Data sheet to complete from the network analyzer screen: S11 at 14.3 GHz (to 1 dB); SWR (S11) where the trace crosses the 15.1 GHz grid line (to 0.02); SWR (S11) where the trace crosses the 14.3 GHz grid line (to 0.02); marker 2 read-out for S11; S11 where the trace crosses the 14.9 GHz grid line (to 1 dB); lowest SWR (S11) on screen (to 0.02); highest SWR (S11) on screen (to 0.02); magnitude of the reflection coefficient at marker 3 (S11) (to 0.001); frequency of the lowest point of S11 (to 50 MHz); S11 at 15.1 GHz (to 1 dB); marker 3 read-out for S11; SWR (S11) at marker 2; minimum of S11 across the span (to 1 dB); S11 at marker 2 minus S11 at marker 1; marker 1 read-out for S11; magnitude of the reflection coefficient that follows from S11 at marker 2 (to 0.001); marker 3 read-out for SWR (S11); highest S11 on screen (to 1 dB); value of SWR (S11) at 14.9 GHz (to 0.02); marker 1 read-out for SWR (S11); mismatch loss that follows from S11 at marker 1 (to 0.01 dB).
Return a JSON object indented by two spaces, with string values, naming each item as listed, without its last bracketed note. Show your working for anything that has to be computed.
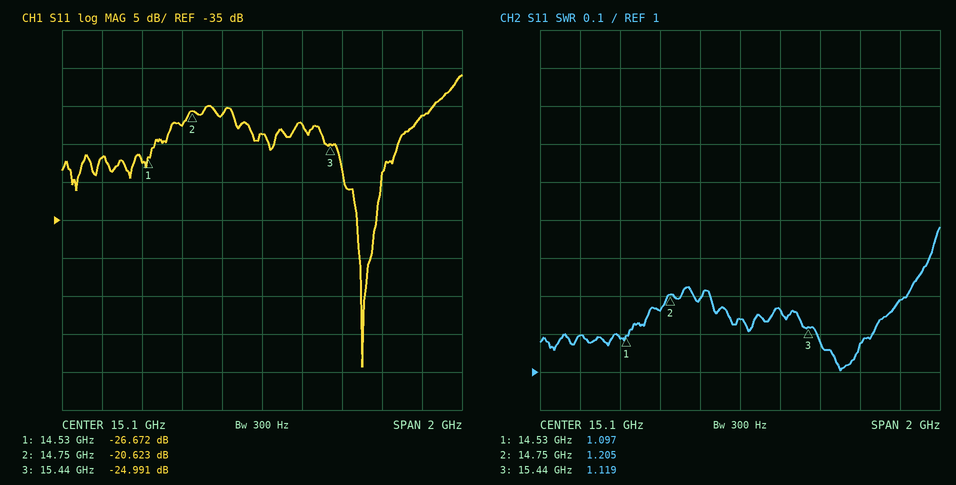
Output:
{
  "S11 at 14.3 GHz": "-27 dB",
  "SWR (S11) where the trace crosses the 15.1 GHz grid line": "1.14",
  "SWR (S11) where the trace crosses the 14.3 GHz grid line": "1.10",
  "marker 2 read-out for S11": "-20.623 dB",
  "S11 where the trace crosses the 14.9 GHz grid line": "-21 dB",
  "lowest SWR (S11) on screen": "1.00",
  "highest SWR (S11) on screen": "1.38",
  "magnitude of the reflection coefficient at marker 3 (S11)": "10^(-24.991/20) ≈ 0.056",
  "frequency of the lowest point of S11": "15.60 GHz",
  "S11 at 15.1 GHz": "-24 dB",
  "marker 3 read-out for S11": "-24.991 dB",
  "SWR (S11) at marker 2": "1.205",
  "minimum of S11 across the span": "-54 dB",
  "S11 at marker 2 minus S11 at marker 1": "-20.623 − (-26.672) = 6.049 dB",
  "marker 1 read-out for S11": "-26.672 dB",
  "magnitude of the reflection coefficient that follows from S11 at marker 2": "10^(-20.623/20) ≈ 0.093",
  "marker 3 read-out for SWR": "1.119",
  "highest S11 on screen": "-16 dB",
  "value of SWR (S11) at 14.9 GHz": "1.20",
  "marker 1 read-out for SWR": "1.097",
  "mismatch loss that follows from S11 at marker 1": "−10 log10(1 − 10^(-26.672/10)) ≈ 0.01 dB"
}
